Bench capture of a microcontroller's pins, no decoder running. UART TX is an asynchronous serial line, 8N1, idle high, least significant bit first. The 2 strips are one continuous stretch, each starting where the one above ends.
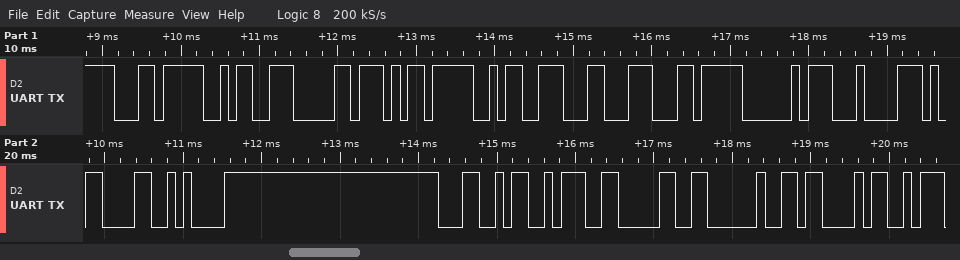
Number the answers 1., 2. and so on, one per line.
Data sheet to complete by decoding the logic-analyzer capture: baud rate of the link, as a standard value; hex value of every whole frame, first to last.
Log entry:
1. 9600 baud
2. EC 9A B0 ED 9A 8C EC A0 84 0D 0A 4C 3A 30 20 43
